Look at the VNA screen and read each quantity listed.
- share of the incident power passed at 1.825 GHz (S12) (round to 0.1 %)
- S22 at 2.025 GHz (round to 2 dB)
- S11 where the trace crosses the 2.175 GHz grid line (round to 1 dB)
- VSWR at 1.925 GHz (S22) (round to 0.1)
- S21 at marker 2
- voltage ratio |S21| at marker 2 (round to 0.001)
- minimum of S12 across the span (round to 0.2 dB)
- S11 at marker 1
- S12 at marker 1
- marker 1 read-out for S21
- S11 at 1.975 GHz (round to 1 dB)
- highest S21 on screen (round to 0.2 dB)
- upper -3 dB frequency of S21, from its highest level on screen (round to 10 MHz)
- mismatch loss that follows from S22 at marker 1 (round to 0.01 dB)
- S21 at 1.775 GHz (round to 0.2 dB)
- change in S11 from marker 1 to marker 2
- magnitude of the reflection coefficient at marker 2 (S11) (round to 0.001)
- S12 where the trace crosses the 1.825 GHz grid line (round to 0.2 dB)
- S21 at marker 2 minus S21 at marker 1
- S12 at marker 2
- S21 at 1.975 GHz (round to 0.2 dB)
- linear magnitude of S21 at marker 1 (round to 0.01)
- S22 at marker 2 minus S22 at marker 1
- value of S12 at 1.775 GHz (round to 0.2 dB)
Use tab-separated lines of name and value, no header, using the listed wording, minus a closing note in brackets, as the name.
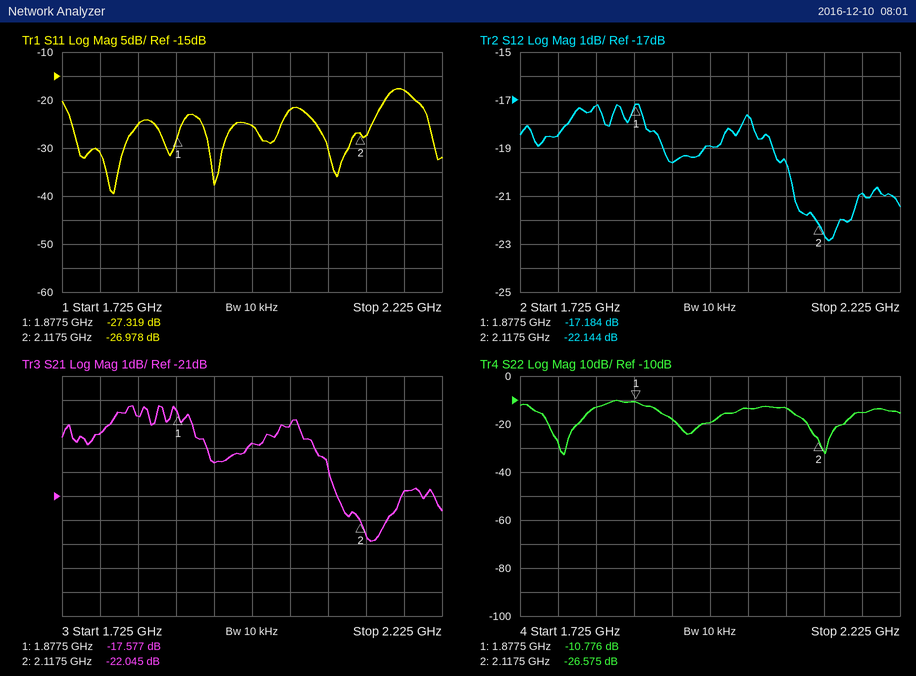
share of the incident power passed at 1.825 GHz (S12)	1.9 %
S22 at 2.025 GHz	-14 dB
S11 where the trace crosses the 2.175 GHz grid line	-18 dB
VSWR at 1.925 GHz (S22)	1.3
S21 at marker 2	-22.045 dB
voltage ratio |S21| at marker 2	0.079
minimum of S12 across the span	-22.8 dB
S11 at marker 1	-27.319 dB
S12 at marker 1	-17.184 dB
marker 1 read-out for S21	-17.577 dB
S11 at 1.975 GHz	-25 dB
highest S21 on screen	-17.2 dB
upper -3 dB frequency of S21, from its highest level on screen	2.08 GHz
mismatch loss that follows from S22 at marker 1	0.38 dB
S21 at 1.775 GHz	-18.4 dB
change in S11 from marker 1 to marker 2	0.341 dB
magnitude of the reflection coefficient at marker 2 (S11)	0.045
S12 where the trace crosses the 1.825 GHz grid line	-17.2 dB
S21 at marker 2 minus S21 at marker 1	-4.468 dB
S12 at marker 2	-22.144 dB
S21 at 1.975 GHz	-18.8 dB
linear magnitude of S21 at marker 1	0.13
S22 at marker 2 minus S22 at marker 1	-15.799 dB
value of S12 at 1.775 GHz	-18.4 dB
